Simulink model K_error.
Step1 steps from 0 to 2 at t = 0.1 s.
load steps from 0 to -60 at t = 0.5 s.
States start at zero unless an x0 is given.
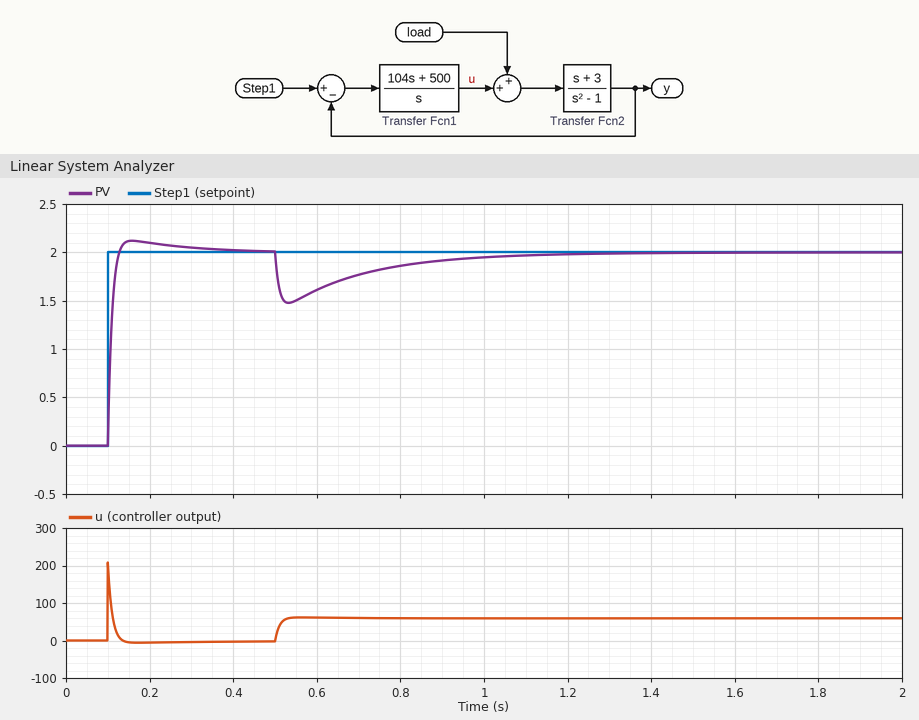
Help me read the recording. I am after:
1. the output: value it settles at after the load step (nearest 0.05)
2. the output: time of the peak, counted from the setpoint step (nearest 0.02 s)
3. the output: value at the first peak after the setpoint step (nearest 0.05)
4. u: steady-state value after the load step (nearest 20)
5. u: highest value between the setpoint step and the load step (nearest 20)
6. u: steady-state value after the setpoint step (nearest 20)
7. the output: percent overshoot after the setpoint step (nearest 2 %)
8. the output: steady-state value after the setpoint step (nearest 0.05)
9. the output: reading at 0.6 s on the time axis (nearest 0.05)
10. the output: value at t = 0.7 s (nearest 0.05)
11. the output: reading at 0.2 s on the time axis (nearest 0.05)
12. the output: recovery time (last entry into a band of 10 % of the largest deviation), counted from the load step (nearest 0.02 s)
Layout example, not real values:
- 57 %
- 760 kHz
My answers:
- 2.00
- 0.06 s
- 2.10
- 60
- 200
- 0
- 6 %
- 2.00
- 1.60
- 1.75
- 2.10
- 0.50 s
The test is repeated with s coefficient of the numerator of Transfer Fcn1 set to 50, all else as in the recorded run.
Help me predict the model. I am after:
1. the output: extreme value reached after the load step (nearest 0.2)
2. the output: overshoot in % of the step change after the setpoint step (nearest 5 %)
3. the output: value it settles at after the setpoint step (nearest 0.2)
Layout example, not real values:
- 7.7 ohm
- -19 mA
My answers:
- 1.0
- 15 %
- 2.0
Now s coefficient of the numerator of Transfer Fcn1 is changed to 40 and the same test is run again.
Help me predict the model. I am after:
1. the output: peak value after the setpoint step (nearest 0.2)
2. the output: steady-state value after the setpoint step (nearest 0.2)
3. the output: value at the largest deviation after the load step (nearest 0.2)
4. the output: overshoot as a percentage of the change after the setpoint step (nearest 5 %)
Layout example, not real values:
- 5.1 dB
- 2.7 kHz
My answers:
- 2.4
- 2.0
- 0.8
- 20 %
